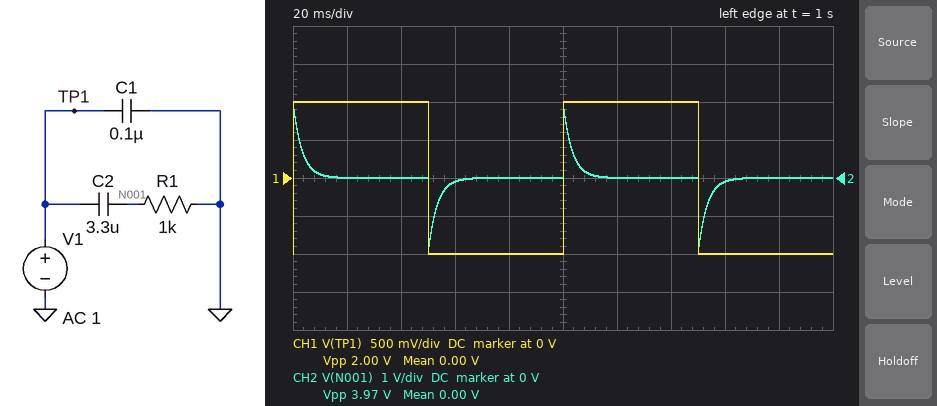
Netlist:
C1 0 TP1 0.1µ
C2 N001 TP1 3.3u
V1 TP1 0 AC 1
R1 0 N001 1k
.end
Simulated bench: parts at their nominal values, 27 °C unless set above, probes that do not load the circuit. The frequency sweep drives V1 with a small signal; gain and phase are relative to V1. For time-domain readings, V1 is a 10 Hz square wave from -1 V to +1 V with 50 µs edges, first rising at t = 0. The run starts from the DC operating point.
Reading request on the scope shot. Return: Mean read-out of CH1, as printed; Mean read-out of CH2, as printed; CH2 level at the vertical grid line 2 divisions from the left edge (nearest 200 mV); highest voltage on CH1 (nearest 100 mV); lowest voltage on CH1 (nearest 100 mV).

0.00 V
0.00 V
0 V
1.0 V
-1.0 V
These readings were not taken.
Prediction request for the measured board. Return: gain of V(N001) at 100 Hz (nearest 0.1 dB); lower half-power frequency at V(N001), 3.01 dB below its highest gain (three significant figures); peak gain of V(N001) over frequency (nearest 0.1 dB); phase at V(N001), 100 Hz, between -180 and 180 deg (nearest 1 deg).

-0.9 dB
48.2 Hz
0 dB
26 deg
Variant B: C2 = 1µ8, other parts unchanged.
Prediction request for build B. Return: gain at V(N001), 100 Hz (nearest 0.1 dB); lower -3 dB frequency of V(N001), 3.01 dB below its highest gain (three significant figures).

-2.5 dB
88.4 Hz
